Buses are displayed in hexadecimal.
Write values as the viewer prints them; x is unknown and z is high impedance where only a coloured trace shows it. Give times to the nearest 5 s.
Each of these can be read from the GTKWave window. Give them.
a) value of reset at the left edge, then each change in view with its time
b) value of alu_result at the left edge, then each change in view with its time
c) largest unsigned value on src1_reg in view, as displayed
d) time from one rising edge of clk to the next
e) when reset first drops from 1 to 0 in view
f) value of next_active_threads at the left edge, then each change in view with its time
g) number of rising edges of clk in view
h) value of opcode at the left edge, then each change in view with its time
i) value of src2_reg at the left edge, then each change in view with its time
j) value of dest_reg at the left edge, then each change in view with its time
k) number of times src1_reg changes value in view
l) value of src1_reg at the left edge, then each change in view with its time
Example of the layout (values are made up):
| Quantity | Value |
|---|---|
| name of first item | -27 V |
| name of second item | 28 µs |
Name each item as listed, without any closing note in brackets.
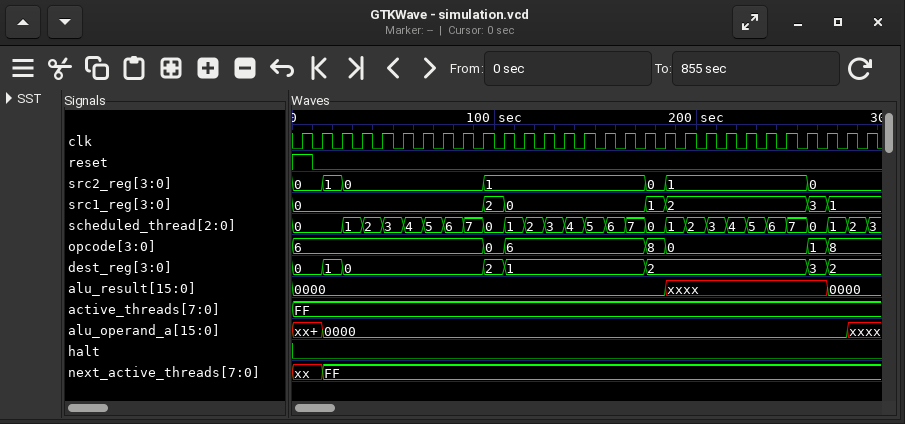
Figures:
| Quantity | Value |
|---|---|
| value of reset at the left edge, then each change in view with its time | 1, 0 at 10 s |
| value of alu_result at the left edge, then each change in view with its time | 0000, xxxx at 185 s, 0000 at 265 s |
| largest unsigned value on src1_reg in view, as displayed | 3 |
| time from one rising edge of clk to the next | 10 s |
| when reset first drops from 1 to 0 in view | 10 s |
| value of next_active_threads at the left edge, then each change in view with its time | xx, FF at 15 s |
| number of rising edges of clk in view | 29 |
| value of opcode at the left edge, then each change in view with its time | 6, 0 at 95 s, 6 at 105 s, 8 at 175 s, 0 at 185 s, 1 at 255 s, 8 at 265 s |
| value of src2_reg at the left edge, then each change in view with its time | 0, 1 at 15 s, 0 at 25 s, 1 at 95 s, 0 at 175 s, 1 at 185 s, 0 at 255 s |
| value of dest_reg at the left edge, then each change in view with its time | 0, 1 at 15 s, 0 at 25 s, 2 at 95 s, 1 at 105 s, 2 at 175 s, 3 at 255 s, 2 at 265 s |
| number of times src1_reg changes value in view | 6 |
| value of src1_reg at the left edge, then each change in view with its time | 0, 2 at 95 s, 0 at 105 s, 1 at 175 s, 2 at 185 s, 3 at 255 s, 1 at 265 s |
